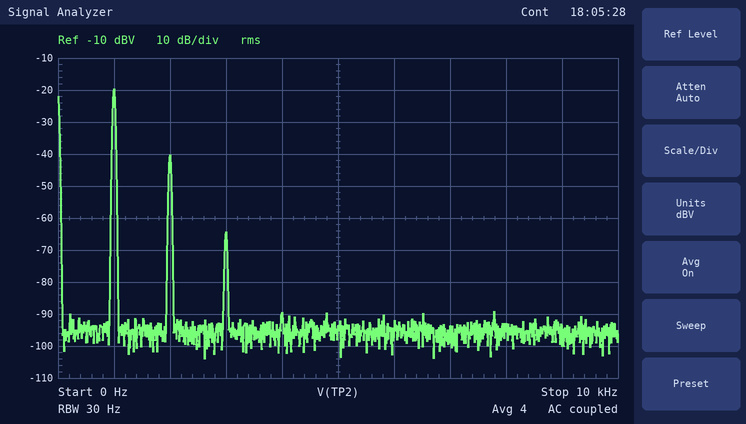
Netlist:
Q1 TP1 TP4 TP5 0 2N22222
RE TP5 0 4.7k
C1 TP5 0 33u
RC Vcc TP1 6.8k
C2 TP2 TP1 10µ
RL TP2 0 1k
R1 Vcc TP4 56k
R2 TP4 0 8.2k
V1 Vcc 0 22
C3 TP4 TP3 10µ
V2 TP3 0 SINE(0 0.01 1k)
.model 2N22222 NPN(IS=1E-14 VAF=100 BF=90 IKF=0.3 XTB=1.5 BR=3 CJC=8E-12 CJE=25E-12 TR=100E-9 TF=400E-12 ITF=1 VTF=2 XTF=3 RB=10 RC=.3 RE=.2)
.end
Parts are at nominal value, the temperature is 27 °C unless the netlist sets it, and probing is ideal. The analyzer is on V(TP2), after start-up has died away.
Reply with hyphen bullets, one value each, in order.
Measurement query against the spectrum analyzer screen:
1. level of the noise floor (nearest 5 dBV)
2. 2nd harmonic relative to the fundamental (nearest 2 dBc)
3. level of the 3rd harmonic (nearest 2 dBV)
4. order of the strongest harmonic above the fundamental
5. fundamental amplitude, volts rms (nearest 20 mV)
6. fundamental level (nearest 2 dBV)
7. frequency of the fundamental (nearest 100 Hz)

- -95 dBV
- -20 dBc
- -64 dBV
- 2
- 100 mV
- -20 dBV
- 1.0 kHz
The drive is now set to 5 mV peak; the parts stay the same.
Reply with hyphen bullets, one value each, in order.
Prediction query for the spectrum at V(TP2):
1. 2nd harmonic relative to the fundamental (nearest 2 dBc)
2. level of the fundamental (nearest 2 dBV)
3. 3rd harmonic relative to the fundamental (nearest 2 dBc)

- -26 dBc
- -26 dBV
- -56 dBc
